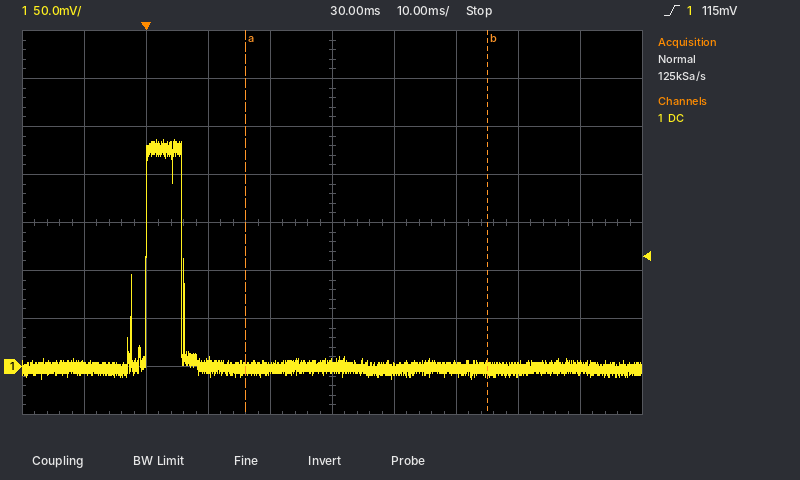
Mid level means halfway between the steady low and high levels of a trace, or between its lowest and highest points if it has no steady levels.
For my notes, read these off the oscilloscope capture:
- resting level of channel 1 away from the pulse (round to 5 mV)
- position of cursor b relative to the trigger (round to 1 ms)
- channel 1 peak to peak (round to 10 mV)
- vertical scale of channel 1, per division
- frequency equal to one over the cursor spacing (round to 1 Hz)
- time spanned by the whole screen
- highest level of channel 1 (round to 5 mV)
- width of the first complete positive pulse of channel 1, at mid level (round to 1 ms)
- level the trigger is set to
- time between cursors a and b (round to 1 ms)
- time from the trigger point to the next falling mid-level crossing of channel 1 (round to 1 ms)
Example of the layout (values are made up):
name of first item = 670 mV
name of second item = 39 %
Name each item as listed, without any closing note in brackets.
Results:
resting level of channel 1 away from the pulse = 0 mV
position of cursor b relative to the trigger = +55 ms
channel 1 peak to peak = 250 mV
vertical scale of channel 1, per division = 50 mV
frequency equal to one over the cursor spacing = 26 Hz
time spanned by the whole screen = 100 ms
highest level of channel 1 = 235 mV
width of the first complete positive pulse of channel 1, at mid level = 6 ms
level the trigger is set to = 115 mV
time between cursors a and b = 39 ms
time from the trigger point to the next falling mid-level crossing of channel 1 = 6 ms
